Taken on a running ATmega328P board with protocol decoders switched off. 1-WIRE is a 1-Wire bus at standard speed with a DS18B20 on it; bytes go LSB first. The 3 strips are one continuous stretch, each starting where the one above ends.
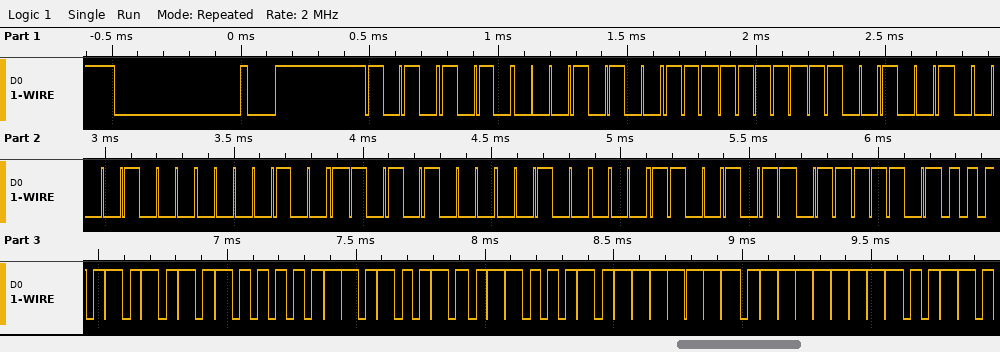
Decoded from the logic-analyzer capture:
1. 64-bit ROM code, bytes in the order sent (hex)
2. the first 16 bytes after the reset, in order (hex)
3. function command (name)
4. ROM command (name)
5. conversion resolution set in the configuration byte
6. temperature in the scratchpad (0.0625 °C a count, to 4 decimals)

28 FF 93 10 90 15 04 D3
55 28 FF 93 10 90 15 04 D3 BE 50 05 4B 46 7F FF
Read Scratchpad
Match ROM
12 bits
85.0000 °C
